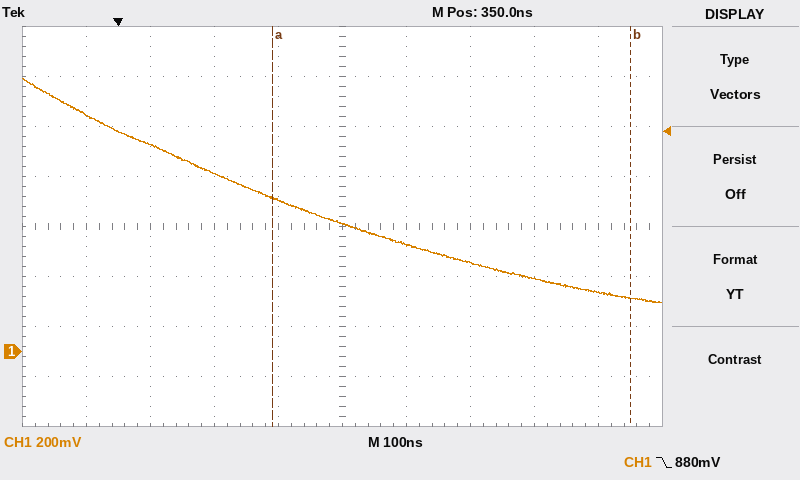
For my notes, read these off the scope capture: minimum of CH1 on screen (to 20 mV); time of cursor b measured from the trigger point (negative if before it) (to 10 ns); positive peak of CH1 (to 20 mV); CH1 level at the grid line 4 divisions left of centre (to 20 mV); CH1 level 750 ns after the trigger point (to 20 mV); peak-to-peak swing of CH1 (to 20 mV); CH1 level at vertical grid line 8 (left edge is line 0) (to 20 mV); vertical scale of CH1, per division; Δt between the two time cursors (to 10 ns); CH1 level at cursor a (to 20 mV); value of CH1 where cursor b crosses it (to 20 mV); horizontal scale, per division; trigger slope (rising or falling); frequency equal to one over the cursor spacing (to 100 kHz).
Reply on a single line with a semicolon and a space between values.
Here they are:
200 mV; +800 ns; 1.10 V; 940 mV; 240 mV; 900 mV; 300 mV; 200 mV; 560 ns; 620 mV; 220 mV; 100 ns; falling; 1.8 MHz
